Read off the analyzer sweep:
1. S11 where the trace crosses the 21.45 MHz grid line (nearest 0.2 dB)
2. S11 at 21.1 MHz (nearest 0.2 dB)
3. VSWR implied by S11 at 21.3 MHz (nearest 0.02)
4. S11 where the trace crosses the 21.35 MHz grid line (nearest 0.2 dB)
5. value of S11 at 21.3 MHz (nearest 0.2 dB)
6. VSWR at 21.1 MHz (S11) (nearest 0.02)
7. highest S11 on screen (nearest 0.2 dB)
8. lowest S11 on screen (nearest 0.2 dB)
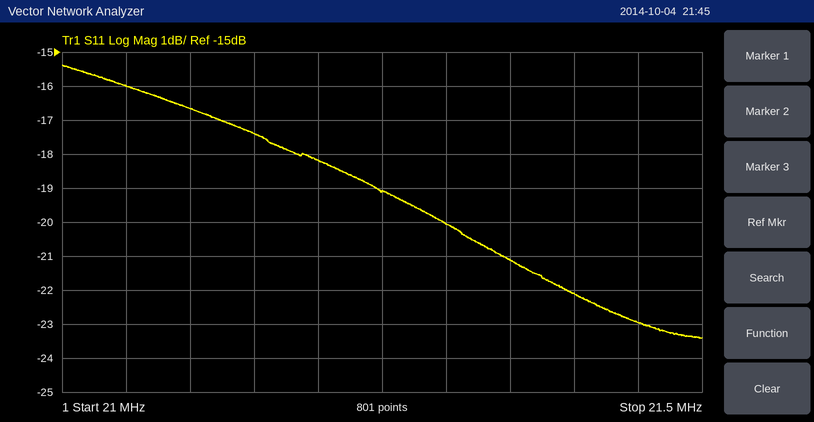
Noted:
-23.0 dB
-16.6 dB
1.22
-21.2 dB
-20.0 dB
1.34
-15.4 dB
-23.4 dB
